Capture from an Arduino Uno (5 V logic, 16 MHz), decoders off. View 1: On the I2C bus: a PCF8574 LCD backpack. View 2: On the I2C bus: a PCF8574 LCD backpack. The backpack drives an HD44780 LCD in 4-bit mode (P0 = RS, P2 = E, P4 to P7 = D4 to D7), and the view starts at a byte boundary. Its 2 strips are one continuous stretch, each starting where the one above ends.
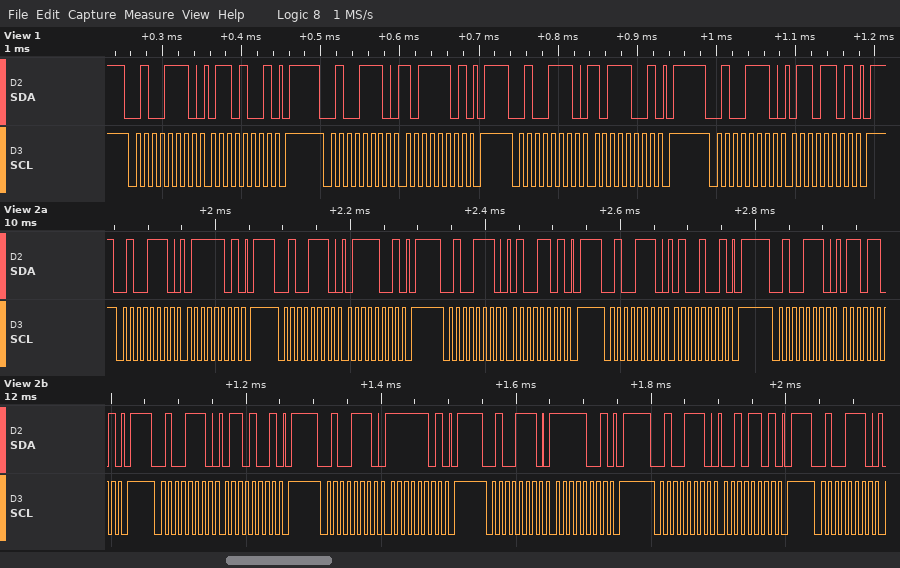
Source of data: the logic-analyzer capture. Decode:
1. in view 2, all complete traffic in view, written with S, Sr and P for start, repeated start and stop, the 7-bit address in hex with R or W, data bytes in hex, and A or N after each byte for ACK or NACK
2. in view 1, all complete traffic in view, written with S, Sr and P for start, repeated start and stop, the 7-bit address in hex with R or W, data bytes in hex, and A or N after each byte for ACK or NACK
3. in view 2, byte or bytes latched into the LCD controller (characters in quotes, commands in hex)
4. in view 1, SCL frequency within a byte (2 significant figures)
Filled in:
S 27W A 7D A P S 27W A 79 A P S 27W A 4D A P S 27W A 49 A P S 27W A 6D A P S 27W A 69 A P S 27W A FD A P S 27W A F9 A P S 27W A 2D A P S 27W A
S 27W A 69 A P S 27W A BD A P S 27W A B9 A P S 27W A 6D A P
't' 'o'
100 kHz
